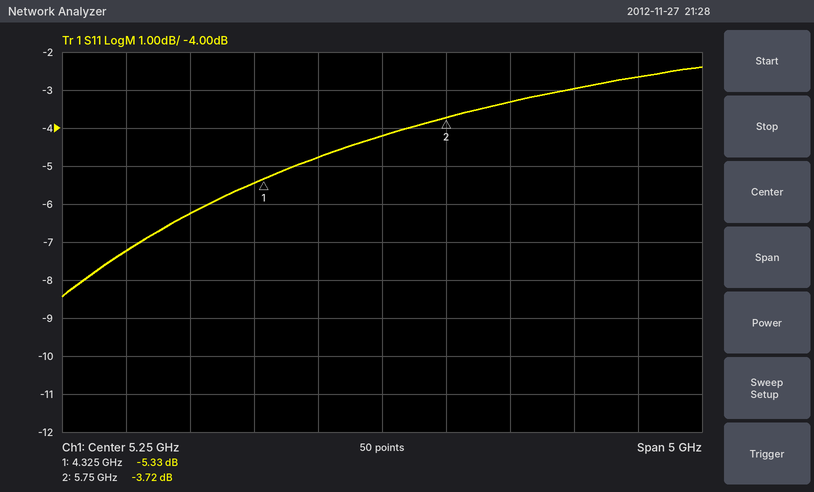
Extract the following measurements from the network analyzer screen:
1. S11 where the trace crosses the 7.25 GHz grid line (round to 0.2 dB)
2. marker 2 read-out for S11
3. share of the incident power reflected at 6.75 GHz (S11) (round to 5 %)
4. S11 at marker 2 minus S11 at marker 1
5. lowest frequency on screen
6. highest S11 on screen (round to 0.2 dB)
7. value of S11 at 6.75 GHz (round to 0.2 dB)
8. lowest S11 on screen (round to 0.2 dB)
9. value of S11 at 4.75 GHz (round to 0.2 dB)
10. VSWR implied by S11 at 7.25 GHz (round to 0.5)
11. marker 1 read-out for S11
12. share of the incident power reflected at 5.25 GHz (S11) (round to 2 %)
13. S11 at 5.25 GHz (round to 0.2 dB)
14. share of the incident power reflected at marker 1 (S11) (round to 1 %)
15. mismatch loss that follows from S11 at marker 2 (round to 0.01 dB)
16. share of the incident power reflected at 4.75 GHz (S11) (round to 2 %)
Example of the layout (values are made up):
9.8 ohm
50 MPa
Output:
-2.6 dB
-3.72 dB
50 %
1.61 dB
2.75 GHz
-2.4 dB
-3.0 dB
-8.4 dB
-4.8 dB
6.5
-5.33 dB
38 %
-4.2 dB
29 %
2.40 dB
34 %
